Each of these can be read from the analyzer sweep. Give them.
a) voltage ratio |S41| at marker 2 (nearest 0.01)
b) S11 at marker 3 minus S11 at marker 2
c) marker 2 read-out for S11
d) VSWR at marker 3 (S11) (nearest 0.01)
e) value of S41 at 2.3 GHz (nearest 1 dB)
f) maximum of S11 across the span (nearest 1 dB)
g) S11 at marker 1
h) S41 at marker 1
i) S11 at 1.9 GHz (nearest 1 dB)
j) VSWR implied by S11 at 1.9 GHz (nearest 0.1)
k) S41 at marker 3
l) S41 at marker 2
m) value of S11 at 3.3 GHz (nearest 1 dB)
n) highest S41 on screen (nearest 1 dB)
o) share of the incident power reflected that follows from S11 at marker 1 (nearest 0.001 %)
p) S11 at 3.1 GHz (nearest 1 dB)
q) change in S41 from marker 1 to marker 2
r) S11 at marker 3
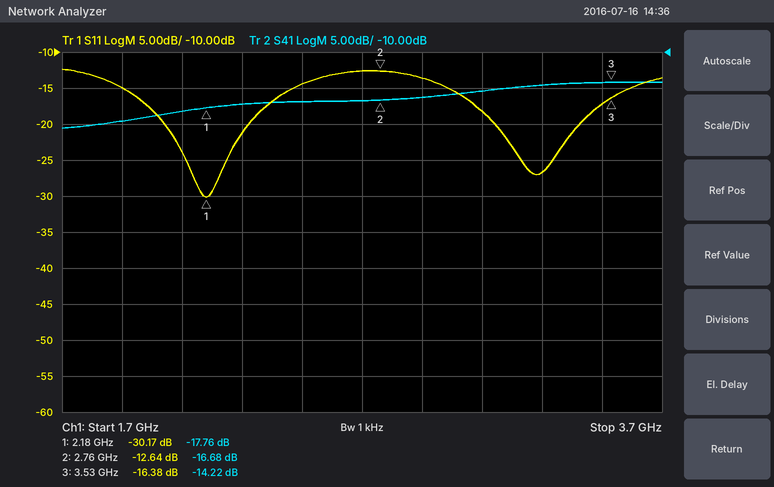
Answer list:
0.15
-3.74 dB
-12.64 dB
1.36
-17 dB
-12 dB
-30.17 dB
-17.76 dB
-15 dB
1.4
-14.22 dB
-16.68 dB
-27 dB
-14 dB
0.096 %
-18 dB
1.08 dB
-16.38 dB
